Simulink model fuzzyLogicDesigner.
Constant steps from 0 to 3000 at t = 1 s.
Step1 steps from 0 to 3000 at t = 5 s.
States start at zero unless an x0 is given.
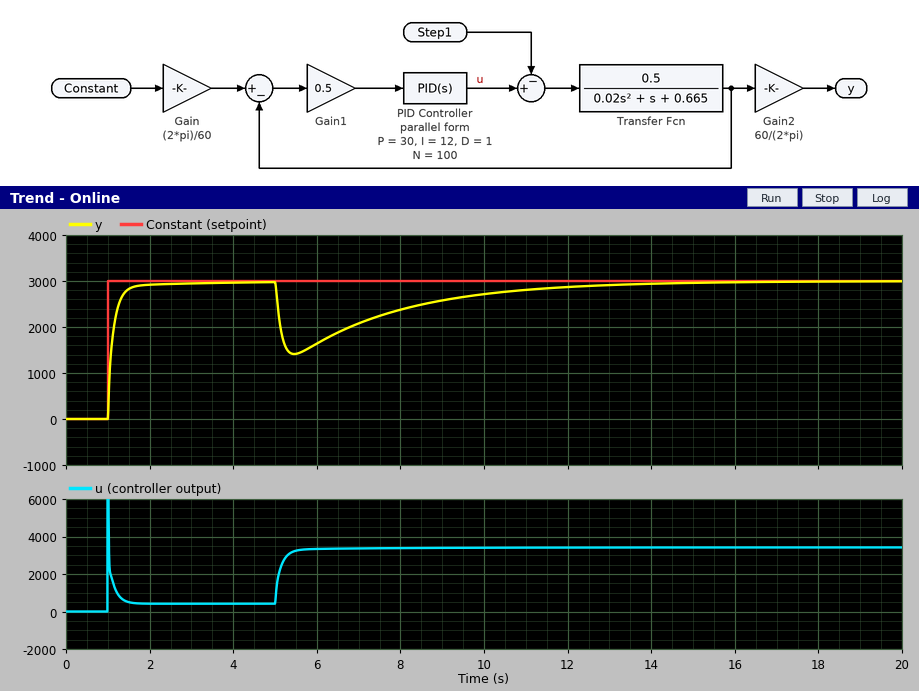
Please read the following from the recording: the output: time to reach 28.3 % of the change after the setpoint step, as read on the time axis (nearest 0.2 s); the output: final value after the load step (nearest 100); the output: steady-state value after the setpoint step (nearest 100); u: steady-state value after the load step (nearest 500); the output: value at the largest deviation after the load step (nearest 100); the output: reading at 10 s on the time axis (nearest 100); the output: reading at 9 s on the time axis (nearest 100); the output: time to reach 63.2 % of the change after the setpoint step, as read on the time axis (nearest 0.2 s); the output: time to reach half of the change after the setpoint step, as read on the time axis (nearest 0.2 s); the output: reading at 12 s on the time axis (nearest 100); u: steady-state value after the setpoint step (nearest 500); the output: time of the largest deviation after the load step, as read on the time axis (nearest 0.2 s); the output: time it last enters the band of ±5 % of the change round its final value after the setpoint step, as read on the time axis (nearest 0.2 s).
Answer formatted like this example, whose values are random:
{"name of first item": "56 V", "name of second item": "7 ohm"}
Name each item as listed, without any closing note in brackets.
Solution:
{"the output: time to reach 28.3 % of the change after the setpoint step, as read on the time axis": "1.0 s", "the output: final value after the load step": "3000", "the output: steady-state value after the setpoint step": "3000", "u: steady-state value after the load step": "3500", "the output: value at the largest deviation after the load step": "1400", "the output: reading at 10 s on the time axis": "2700", "the output: reading at 9 s on the time axis": "2600", "the output: time to reach 63.2 % of the change after the setpoint step, as read on the time axis": "1.2 s", "the output: time to reach half of the change after the setpoint step, as read on the time axis": "1.0 s", "the output: reading at 12 s on the time axis": "2900", "u: steady-state value after the setpoint step": "500", "the output: time of the largest deviation after the load step, as read on the time axis": "5.4 s", "the output: time it last enters the band of ±5 % of the change round its final value after the setpoint step, as read on the time axis": "1.6 s"}
